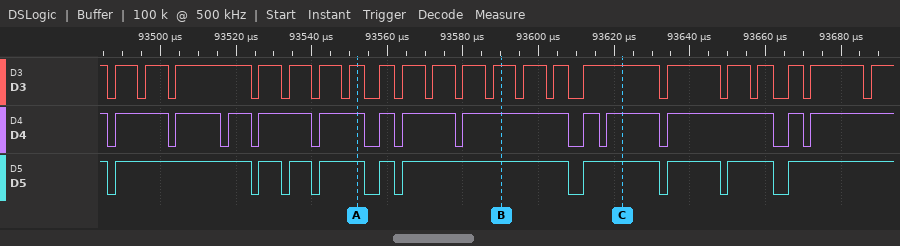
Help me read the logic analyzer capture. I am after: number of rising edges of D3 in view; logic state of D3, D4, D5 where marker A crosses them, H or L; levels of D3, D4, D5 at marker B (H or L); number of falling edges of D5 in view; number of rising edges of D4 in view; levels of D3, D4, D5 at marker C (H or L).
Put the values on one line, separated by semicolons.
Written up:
21; D3=H, D4=H, D5=H; D3=H, D4=H, D5=H; 10; 13; D3=H, D4=H, D5=H
